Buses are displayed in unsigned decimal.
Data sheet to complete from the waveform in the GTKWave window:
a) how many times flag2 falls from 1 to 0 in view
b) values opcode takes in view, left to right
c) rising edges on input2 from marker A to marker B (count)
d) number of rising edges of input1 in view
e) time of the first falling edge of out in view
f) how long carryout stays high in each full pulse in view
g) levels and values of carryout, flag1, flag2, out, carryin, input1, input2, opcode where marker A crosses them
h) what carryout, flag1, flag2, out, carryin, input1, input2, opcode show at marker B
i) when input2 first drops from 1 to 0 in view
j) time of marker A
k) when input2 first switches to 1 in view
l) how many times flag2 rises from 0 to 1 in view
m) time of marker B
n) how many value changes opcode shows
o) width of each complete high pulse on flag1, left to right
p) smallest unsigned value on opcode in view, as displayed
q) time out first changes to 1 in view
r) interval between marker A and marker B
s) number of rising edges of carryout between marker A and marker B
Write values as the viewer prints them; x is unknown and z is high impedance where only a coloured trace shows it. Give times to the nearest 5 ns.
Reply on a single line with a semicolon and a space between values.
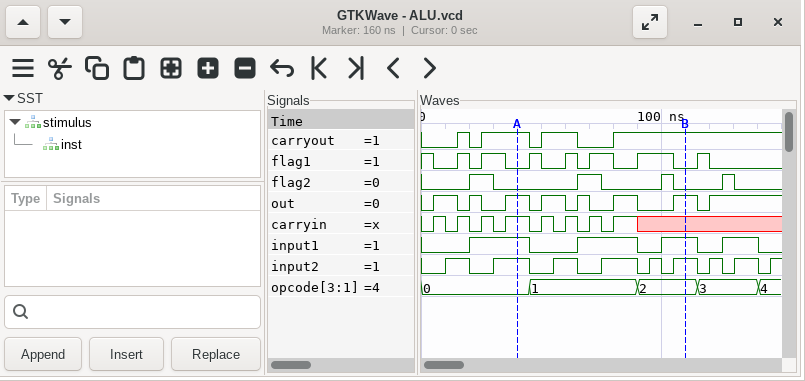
4; 0, 1, 2, 3, 4; 4; 4; 15 ns; 5 ns, 20 ns, 15 ns; carryout=1, flag1=0, flag2=0, out=1, carryin=1, input1=1, input2=1, opcode=0; carryout=1, flag1=0, flag2=0, out=1, carryin=x, input1=1, input2=1, opcode=2; 20 ns; 40 ns; 10 ns; 4; 110 ns; 4; 5 ns, 10 ns, 5 ns, 5 ns, 10 ns, 15 ns, 5 ns; 0; 5 ns; 70 ns; 2
